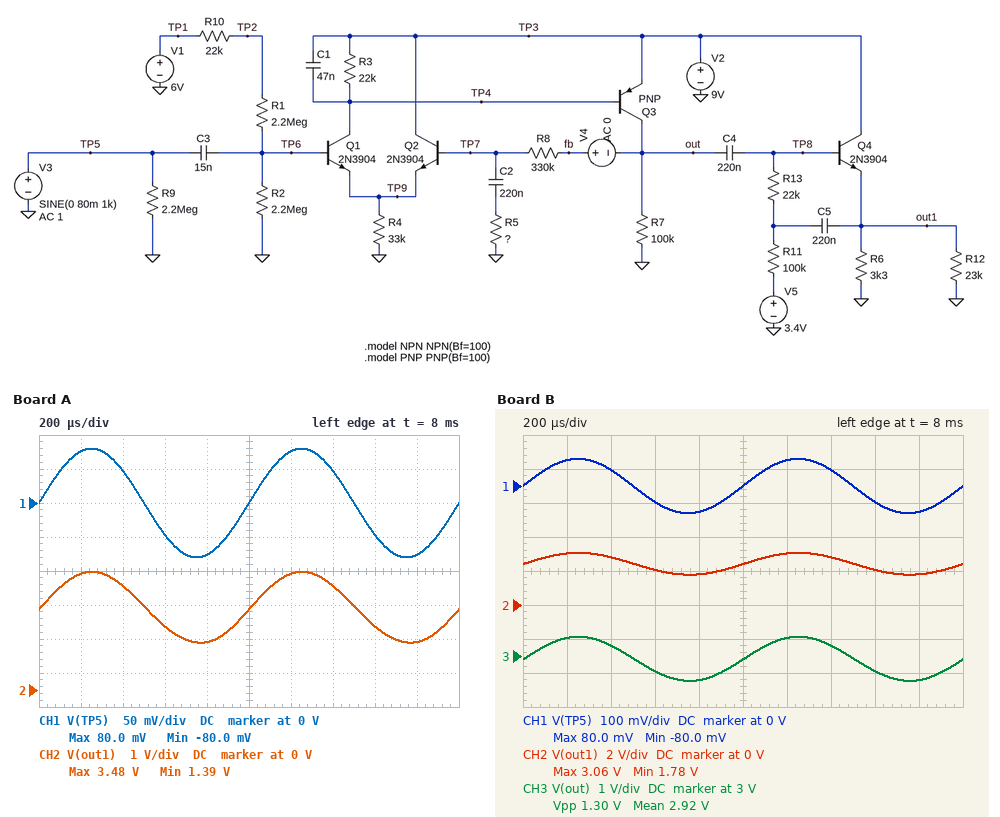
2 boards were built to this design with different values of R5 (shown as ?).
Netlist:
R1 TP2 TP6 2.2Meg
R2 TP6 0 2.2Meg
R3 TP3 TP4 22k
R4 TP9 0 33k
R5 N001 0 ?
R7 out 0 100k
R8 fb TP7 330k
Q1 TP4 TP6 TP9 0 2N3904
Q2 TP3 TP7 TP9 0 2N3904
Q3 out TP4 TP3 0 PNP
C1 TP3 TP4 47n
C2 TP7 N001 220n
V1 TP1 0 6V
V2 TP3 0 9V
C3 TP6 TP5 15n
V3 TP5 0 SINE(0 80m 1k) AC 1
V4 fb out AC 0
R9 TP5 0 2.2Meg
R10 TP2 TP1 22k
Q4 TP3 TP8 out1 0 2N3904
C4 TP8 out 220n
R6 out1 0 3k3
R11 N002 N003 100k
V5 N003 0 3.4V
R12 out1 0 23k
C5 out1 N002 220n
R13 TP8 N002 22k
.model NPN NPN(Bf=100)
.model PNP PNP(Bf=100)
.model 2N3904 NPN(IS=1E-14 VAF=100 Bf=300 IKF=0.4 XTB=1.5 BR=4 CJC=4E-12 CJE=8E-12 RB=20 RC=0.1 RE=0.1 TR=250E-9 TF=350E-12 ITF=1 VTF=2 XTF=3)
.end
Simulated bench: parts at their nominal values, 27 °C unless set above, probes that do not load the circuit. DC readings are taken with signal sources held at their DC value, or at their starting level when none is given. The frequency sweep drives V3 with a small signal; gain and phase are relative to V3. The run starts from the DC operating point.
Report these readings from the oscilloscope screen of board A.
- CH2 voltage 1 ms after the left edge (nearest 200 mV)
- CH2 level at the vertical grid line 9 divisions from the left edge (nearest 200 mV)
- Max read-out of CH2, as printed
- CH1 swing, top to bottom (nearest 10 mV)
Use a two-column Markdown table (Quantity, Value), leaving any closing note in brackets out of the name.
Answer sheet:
| Quantity | Value |
|---|---|
| CH2 voltage 1 ms after the left edge | 2.4 V |
| CH2 level at the vertical grid line 9 divisions from the left edge | 1.4 V |
| Max read-out of CH2, as printed | 3.48 V |
| CH1 swing, top to bottom | 160 mV |
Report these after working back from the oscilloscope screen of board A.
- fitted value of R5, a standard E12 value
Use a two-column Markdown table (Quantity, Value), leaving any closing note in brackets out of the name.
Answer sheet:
| Quantity | Value |
|---|---|
| fitted value of R5, a standard E12 value | 27 kΩ |
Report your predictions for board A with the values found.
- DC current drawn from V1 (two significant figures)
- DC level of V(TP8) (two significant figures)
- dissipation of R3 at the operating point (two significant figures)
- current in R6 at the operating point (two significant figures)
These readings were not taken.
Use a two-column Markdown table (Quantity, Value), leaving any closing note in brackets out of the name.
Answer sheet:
| Quantity | Value |
|---|---|
| DC current drawn from V1 | 1.4 µA |
| DC level of V(TP8) | 3.1 V |
| dissipation of R3 at the operating point | 21 µW |
| current in R6 at the operating point | 740 µA |
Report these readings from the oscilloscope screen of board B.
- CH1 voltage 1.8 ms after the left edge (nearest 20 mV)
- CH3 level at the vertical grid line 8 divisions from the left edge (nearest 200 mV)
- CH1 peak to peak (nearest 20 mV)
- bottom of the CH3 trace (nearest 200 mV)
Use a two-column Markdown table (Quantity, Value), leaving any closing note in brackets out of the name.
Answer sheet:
| Quantity | Value |
|---|---|
| CH1 voltage 1.8 ms after the left edge | -80 mV |
| CH3 level at the vertical grid line 8 divisions from the left edge | 2.6 V |
| CH1 peak to peak | 160 mV |
| bottom of the CH3 trace | 2.2 V |
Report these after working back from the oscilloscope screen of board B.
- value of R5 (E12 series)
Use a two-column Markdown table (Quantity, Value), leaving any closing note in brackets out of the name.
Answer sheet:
| Quantity | Value |
|---|---|
| value of R5 | 47 kΩ |
